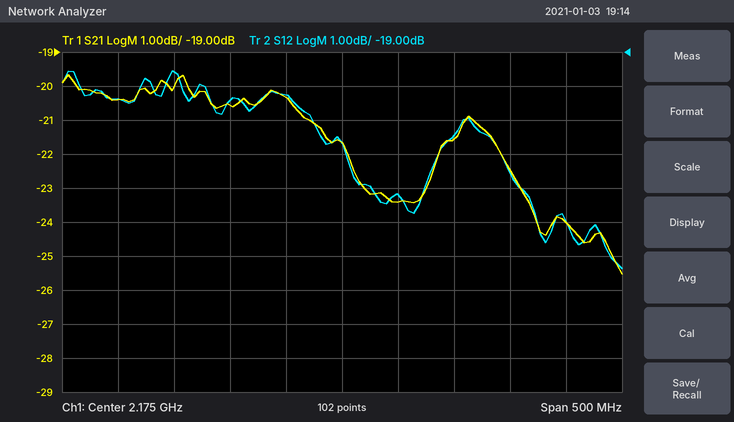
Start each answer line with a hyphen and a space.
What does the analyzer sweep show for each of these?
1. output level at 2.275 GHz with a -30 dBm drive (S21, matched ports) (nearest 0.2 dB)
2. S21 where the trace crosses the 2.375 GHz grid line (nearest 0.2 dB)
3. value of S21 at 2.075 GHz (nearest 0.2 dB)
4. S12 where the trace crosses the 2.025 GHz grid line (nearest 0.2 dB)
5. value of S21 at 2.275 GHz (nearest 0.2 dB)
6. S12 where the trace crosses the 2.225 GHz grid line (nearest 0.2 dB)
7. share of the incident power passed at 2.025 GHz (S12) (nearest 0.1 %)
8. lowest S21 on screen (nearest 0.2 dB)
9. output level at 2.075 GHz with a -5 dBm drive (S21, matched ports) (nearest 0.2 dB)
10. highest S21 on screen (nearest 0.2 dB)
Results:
- -51.6 dBm
- -24.0 dB
- -20.6 dB
- -19.6 dB
- -21.6 dB
- -23.2 dB
- 1.1 %
- -25.6 dB
- -25.6 dBm
- -19.6 dB
